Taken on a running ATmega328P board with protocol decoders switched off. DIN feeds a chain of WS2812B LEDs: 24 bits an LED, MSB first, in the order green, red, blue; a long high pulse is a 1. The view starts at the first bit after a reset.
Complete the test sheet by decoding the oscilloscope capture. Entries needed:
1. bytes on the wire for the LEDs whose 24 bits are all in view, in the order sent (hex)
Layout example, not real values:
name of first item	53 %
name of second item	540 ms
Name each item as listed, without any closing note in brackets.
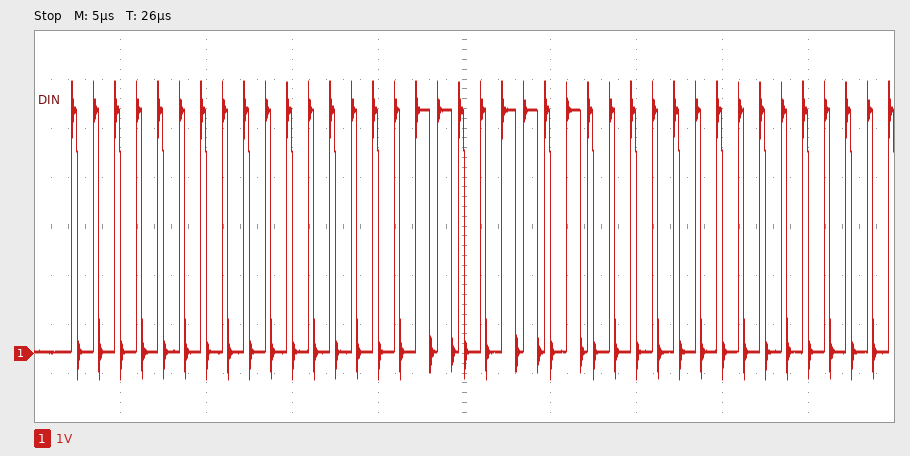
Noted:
bytes on the wire for the LEDs whose 24 bits are all in view, in the order sent	00 00 CD
